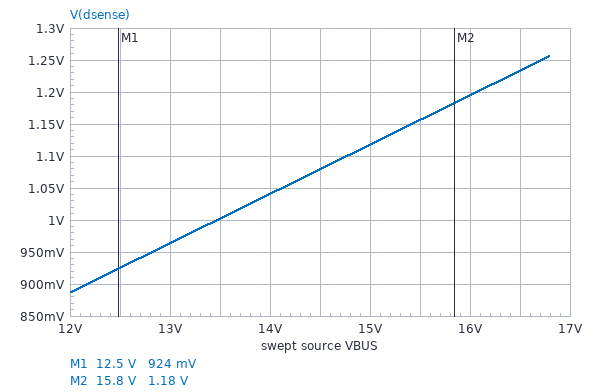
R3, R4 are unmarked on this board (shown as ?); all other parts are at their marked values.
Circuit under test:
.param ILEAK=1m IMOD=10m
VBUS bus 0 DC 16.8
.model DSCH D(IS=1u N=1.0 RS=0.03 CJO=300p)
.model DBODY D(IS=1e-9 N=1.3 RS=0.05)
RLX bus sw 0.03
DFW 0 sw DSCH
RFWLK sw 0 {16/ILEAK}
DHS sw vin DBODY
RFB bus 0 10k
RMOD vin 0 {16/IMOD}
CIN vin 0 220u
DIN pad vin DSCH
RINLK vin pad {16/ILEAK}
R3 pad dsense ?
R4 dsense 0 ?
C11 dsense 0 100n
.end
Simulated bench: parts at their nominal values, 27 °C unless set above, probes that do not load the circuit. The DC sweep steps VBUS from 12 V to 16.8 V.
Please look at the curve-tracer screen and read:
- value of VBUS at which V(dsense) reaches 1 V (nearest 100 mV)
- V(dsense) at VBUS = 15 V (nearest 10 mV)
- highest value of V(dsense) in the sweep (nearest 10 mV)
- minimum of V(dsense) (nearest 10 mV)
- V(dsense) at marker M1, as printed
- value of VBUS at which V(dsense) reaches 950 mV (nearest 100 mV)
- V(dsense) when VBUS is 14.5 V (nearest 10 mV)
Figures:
13.5 V
1.12 V
1.26 V
890 mV
924 mV
12.8 V
1.08 V
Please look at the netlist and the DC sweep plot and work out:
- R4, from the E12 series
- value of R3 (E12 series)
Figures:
8.2 kΩ
82 kΩ
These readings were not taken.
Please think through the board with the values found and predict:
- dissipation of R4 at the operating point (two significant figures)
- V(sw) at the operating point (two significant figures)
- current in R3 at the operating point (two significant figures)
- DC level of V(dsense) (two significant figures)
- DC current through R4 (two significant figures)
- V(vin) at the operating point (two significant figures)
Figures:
190 µW
17 V
150 µA
1.3 V
150 µA
16 V
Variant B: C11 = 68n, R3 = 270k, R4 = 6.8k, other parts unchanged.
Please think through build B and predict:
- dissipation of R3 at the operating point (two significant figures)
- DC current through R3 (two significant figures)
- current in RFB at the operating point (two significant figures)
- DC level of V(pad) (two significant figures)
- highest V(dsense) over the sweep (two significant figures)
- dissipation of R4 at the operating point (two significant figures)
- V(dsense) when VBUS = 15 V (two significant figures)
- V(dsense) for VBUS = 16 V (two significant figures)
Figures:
830 µW
56 µA
1.7 mA
15 V
380 mV
21 µW
340 mV
360 mV
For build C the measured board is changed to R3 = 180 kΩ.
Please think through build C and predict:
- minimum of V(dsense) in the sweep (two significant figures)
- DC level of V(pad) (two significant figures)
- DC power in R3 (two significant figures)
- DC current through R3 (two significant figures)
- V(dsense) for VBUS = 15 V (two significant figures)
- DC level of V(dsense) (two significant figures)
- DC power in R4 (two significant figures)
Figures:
460 mV
15 V
1.1 mW
80 µA
580 mV
650 mV
52 µW
